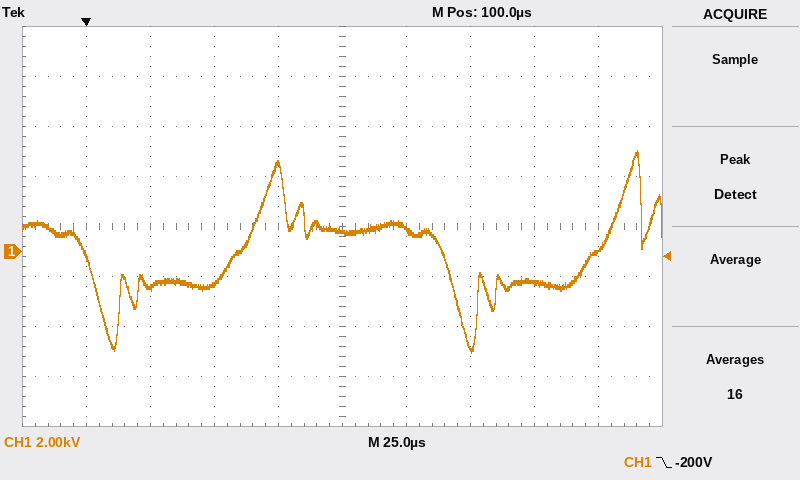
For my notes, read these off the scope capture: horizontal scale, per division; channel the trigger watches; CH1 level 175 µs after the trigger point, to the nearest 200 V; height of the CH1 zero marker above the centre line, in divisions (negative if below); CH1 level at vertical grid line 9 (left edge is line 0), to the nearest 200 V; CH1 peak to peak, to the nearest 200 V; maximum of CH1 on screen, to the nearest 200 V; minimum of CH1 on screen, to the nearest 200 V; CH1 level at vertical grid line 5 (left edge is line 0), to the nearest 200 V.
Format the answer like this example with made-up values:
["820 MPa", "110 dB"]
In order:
["25 µs", "CH1", "-1.2 kV", "-0.5 div", "0.0 kV", "8.0 kV", "4.0 kV", "-4.0 kV", "800 V"]
